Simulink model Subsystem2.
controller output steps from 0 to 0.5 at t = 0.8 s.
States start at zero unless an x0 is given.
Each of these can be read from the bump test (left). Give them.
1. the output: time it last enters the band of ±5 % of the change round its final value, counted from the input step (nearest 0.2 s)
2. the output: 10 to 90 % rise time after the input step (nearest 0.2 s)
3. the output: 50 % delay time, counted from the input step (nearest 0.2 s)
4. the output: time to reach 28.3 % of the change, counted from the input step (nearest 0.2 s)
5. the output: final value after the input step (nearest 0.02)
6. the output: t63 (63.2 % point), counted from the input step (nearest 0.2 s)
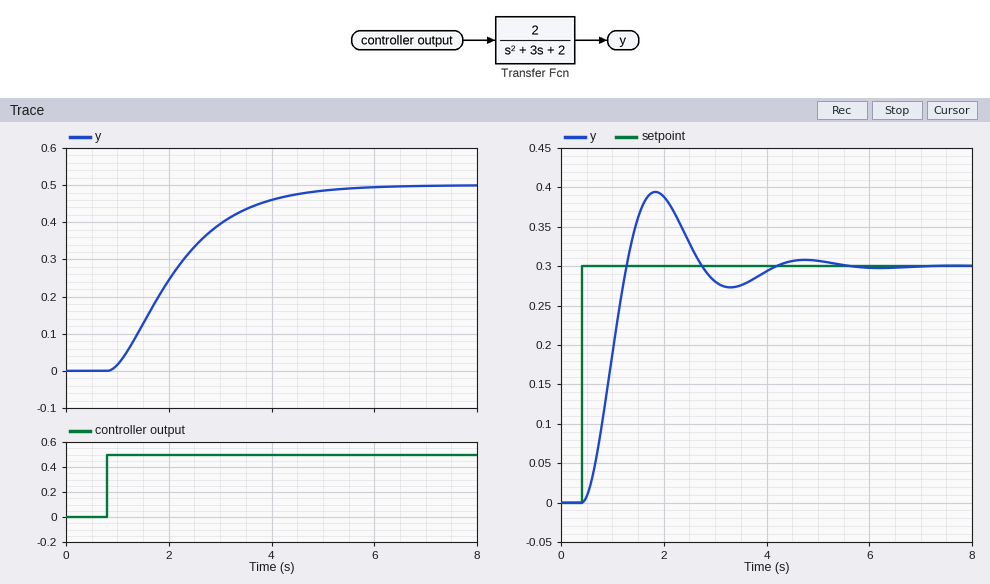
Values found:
3.6 s
2.6 s
1.2 s
0.8 s
0.50
1.6 s
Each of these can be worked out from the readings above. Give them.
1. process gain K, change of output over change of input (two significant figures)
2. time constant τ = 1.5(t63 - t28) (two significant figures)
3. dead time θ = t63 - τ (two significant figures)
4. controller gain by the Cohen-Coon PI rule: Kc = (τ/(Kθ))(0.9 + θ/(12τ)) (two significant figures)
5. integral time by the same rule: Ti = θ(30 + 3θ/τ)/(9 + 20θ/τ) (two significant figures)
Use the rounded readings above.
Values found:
1.0
1.2 s
0.40 s
2.8
0.79 s
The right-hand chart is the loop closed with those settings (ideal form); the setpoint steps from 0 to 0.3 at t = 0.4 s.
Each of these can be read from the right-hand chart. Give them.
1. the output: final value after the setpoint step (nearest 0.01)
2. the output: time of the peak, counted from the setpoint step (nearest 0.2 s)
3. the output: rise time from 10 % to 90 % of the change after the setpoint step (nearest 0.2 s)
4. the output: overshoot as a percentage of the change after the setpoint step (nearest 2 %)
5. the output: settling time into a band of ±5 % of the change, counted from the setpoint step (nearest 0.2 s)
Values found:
0.30
1.4 s
0.6 s
32 %
3.4 s
